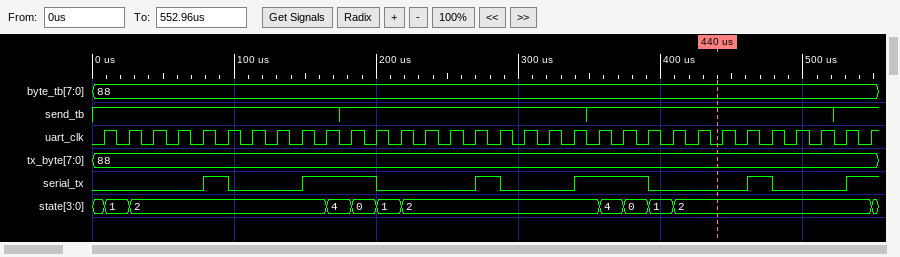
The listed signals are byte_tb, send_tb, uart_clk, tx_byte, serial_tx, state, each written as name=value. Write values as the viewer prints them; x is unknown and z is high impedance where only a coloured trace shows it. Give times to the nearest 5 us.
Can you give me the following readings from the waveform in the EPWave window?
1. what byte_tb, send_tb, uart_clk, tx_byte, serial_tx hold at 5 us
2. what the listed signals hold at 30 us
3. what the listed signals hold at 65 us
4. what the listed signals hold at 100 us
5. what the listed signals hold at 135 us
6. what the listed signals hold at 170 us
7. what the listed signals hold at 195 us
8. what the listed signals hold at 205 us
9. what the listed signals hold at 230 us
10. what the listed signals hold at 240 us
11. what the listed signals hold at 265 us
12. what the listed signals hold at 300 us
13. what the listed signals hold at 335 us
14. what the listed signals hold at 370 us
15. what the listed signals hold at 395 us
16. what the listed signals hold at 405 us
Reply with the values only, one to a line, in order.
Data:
byte_tb=88, send_tb=1, uart_clk=0, tx_byte=88, serial_tx=0
byte_tb=88, send_tb=1, uart_clk=1, tx_byte=88, serial_tx=0, state=2
byte_tb=88, send_tb=1, uart_clk=1, tx_byte=88, serial_tx=0, state=2
byte_tb=88, send_tb=1, uart_clk=1, tx_byte=88, serial_tx=0, state=2
byte_tb=88, send_tb=1, uart_clk=1, tx_byte=88, serial_tx=0, state=2
byte_tb=88, send_tb=1, uart_clk=1, tx_byte=88, serial_tx=1, state=4
byte_tb=88, send_tb=1, uart_clk=0, tx_byte=88, serial_tx=1, state=0
byte_tb=88, send_tb=1, uart_clk=1, tx_byte=88, serial_tx=0, state=1
byte_tb=88, send_tb=1, uart_clk=0, tx_byte=88, serial_tx=0, state=2
byte_tb=88, send_tb=1, uart_clk=1, tx_byte=88, serial_tx=0, state=2
byte_tb=88, send_tb=1, uart_clk=0, tx_byte=88, serial_tx=0, state=2
byte_tb=88, send_tb=1, uart_clk=0, tx_byte=88, serial_tx=0, state=2
byte_tb=88, send_tb=1, uart_clk=0, tx_byte=88, serial_tx=0, state=2
byte_tb=88, send_tb=1, uart_clk=0, tx_byte=88, serial_tx=1, state=4
byte_tb=88, send_tb=1, uart_clk=1, tx_byte=88, serial_tx=0, state=1
byte_tb=88, send_tb=1, uart_clk=0, tx_byte=88, serial_tx=0, state=1
